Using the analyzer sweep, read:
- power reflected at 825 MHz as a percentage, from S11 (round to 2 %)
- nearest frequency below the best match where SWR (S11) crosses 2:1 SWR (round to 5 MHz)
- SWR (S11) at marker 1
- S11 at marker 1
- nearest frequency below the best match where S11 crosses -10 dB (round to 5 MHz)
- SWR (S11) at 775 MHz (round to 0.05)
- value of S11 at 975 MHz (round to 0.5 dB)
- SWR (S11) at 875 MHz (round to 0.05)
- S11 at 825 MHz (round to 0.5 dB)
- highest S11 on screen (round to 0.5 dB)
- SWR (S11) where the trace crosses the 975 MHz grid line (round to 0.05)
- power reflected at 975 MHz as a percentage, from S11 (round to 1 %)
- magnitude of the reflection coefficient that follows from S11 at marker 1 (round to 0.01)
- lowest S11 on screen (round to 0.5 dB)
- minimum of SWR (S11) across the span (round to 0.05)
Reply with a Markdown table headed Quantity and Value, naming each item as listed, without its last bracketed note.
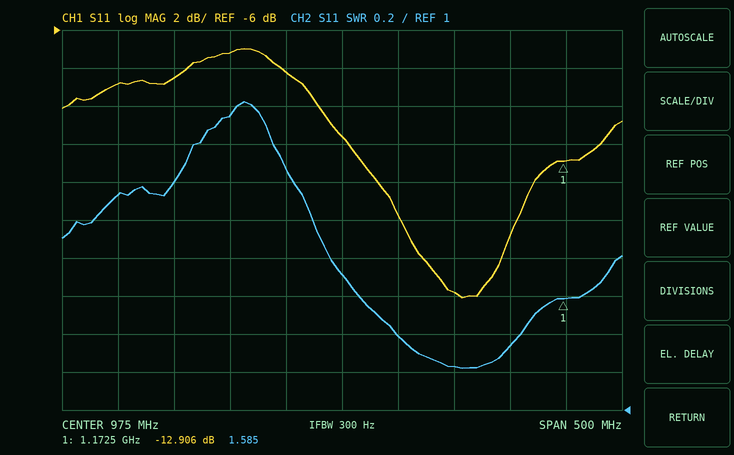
| Quantity | Value |
|---|---|
| power reflected at 825 MHz as a percentage, from S11 | 14 % |
| nearest frequency below the best match where SWR (S11) crosses 2:1 SWR | 950 MHz |
| SWR (S11) at marker 1 | 1.585 |
| S11 at marker 1 | -12.906 dB |
| nearest frequency below the best match where S11 crosses -10 dB | 955 MHz |
| SWR (S11) at 775 MHz | 2.15 |
| value of S11 at 975 MHz | -11.5 dB |
| SWR (S11) at 875 MHz | 2.55 |
| S11 at 825 MHz | -8.5 dB |
| highest S11 on screen | -7.0 dB |
| SWR (S11) where the trace crosses the 975 MHz grid line | 1.70 |
| power reflected at 975 MHz as a percentage, from S11 | 7 % |
| magnitude of the reflection coefficient that follows from S11 at marker 1 | 0.23 |
| lowest S11 on screen | -20.0 dB |
| minimum of SWR (S11) across the span | 1.20 |
